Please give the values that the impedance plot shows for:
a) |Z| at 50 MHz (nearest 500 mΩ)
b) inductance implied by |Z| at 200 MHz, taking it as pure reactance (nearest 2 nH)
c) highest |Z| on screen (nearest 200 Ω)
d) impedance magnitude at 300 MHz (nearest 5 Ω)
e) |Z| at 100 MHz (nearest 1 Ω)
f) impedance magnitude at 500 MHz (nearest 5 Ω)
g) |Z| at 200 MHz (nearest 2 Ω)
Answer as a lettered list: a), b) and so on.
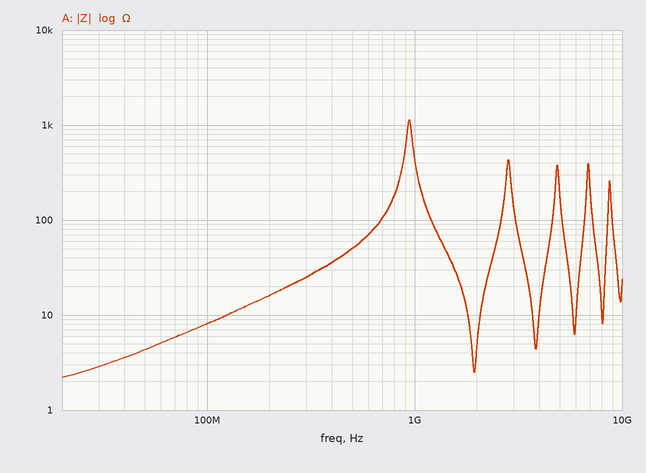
a) 4.5 Ω
b) 12 nH
c) 1.2 kΩ
d) 25 Ω
e) 8 Ω
f) 50 Ω
g) 16 Ω
